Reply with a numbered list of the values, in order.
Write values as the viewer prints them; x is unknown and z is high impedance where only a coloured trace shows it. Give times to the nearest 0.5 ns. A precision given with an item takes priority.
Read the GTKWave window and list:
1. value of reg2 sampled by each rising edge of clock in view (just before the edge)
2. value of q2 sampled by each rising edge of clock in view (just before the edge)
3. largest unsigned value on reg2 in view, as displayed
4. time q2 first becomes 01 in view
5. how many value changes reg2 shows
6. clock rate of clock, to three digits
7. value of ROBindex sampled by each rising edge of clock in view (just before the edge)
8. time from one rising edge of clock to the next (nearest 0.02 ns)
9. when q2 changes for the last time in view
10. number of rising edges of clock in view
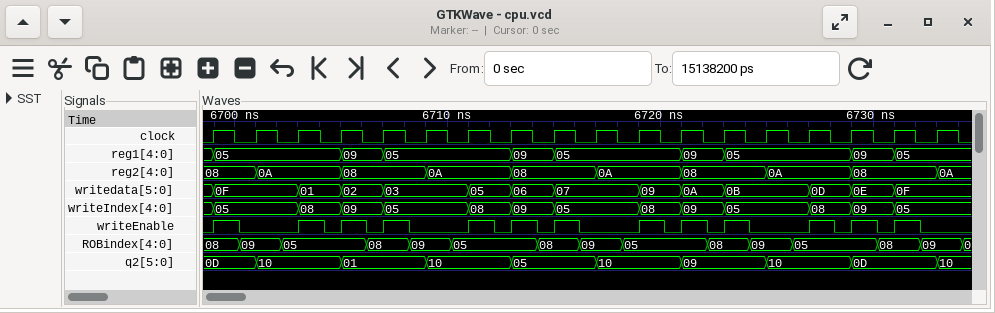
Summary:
1. 08, 08, 0A, 0A, 08, 08, 0A, 0A, 08, 08, 0A, 0A, 08, 08, 0A, 0A, 08, 08
2. 0D, 0D, 10, 10, 01, 01, 10, 10, 05, 05, 10, 10, 09, 09, 10, 10, 0D, 0D
3. 0A
4. 6705 ns
5. 9
6. 500 MHz
7. 08, 09, 05, 05, 08, 09, 05, 05, 08, 09, 05, 05, 08, 09, 05, 05, 08, 09
8. 2 ns
9. 6733 ns
10. 18
